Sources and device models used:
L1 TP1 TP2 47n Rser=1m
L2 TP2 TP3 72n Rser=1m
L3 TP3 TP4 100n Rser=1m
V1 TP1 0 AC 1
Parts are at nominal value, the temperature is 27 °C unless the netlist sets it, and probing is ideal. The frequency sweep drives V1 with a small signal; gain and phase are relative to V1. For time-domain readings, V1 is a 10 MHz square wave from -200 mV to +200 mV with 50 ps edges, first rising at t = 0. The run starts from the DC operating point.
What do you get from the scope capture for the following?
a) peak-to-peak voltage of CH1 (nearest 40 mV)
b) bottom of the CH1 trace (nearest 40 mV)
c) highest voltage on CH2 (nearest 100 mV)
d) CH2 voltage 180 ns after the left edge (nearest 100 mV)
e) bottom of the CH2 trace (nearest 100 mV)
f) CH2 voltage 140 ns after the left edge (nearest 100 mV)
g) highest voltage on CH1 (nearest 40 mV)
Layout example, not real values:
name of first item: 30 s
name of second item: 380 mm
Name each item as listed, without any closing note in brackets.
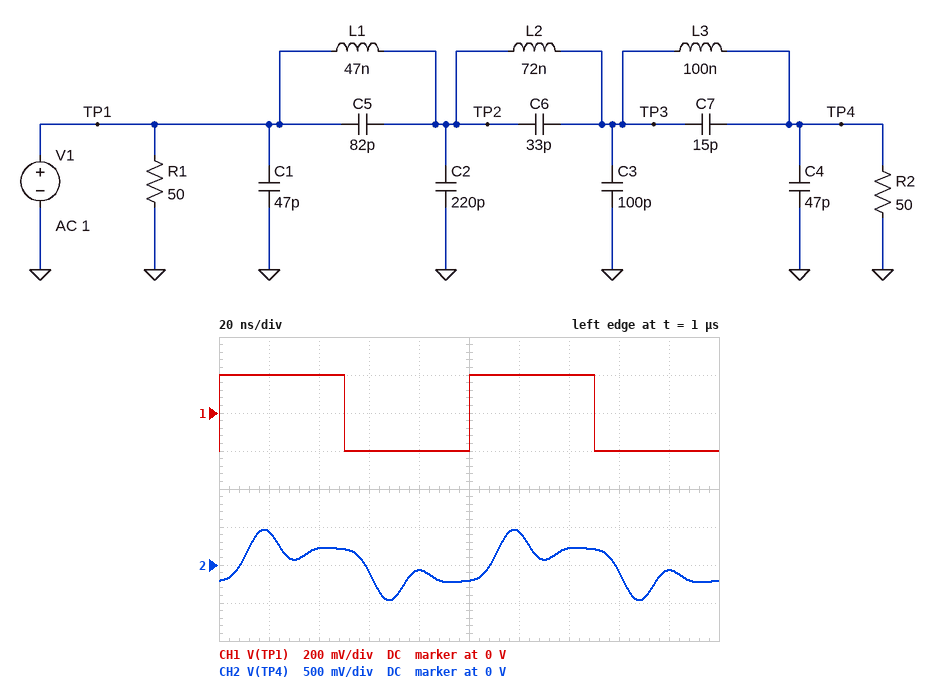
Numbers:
peak-to-peak voltage of CH1: 400 mV
bottom of the CH1 trace: -200 mV
highest voltage on CH2: 500 mV
CH2 voltage 180 ns after the left edge: -100 mV
bottom of the CH2 trace: -500 mV
CH2 voltage 140 ns after the left edge: 200 mV
highest voltage on CH1: 200 mV
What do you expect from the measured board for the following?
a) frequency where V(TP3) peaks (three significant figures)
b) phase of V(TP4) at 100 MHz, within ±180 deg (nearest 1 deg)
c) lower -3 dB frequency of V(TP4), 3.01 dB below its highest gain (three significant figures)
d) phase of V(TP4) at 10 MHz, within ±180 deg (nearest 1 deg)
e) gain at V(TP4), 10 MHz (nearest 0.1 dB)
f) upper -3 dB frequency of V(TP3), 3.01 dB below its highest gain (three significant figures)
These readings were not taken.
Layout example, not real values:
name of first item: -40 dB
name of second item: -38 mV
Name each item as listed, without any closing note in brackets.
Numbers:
frequency where V(TP3) peaks: 33.3 MHz
phase of V(TP4) at 100 MHz, within ±180 deg: 42 deg
lower -3 dB frequency of V(TP4), 3.01 dB below its highest gain: 22.5 MHz
phase of V(TP4) at 10 MHz, within ±180 deg: -17 deg
gain at V(TP4), 10 MHz: 0.8 dB
upper -3 dB frequency of V(TP3), 3.01 dB below its highest gain: 47.9 MHz
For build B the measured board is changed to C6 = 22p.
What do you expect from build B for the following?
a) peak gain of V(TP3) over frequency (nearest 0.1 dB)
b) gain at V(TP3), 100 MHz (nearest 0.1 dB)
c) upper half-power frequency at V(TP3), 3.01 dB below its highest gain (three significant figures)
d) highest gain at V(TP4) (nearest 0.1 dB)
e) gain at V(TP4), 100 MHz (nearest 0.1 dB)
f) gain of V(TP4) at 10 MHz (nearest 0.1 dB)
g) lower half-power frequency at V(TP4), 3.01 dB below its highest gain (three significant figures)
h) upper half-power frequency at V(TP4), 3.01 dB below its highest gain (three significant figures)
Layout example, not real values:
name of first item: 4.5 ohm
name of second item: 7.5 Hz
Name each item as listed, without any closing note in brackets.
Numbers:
peak gain of V(TP3) over frequency: 6.3 dB
gain at V(TP3), 100 MHz: -33.4 dB
upper half-power frequency at V(TP3), 3.01 dB below its highest gain: 46.6 MHz
highest gain at V(TP4): 7.3 dB
gain at V(TP4), 100 MHz: -46.9 dB
gain of V(TP4) at 10 MHz: 0.8 dB
lower half-power frequency at V(TP4), 3.01 dB below its highest gain: 22.8 MHz
upper half-power frequency at V(TP4), 3.01 dB below its highest gain: 47.5 MHz
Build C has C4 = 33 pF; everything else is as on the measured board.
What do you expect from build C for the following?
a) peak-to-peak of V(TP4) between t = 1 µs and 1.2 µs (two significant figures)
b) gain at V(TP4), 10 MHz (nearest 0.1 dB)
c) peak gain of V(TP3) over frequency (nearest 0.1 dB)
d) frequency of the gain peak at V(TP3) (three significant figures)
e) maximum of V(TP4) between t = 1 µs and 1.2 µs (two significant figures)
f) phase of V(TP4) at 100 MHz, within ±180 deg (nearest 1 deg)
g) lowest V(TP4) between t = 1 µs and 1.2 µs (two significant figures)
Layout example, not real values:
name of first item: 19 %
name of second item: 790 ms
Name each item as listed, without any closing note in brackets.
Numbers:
peak-to-peak of V(TP4) between t = 1 µs and 1.2 µs: 890 mV
gain at V(TP4), 10 MHz: 0.7 dB
peak gain of V(TP3) over frequency: 7.3 dB
frequency of the gain peak at V(TP3): 35.5 MHz
maximum of V(TP4) between t = 1 µs and 1.2 µs: 450 mV
phase of V(TP4) at 100 MHz, within ±180 deg: 56 deg
lowest V(TP4) between t = 1 µs and 1.2 µs: -450 mV
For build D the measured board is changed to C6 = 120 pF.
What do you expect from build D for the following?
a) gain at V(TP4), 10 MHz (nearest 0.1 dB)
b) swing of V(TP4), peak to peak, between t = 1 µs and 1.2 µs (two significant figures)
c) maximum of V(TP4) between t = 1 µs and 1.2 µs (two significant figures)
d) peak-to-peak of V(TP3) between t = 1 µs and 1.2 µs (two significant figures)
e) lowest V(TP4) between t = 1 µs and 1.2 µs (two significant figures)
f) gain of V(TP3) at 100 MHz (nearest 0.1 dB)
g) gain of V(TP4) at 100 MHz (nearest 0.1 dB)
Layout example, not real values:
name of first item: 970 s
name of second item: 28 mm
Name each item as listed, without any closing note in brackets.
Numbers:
gain at V(TP4), 10 MHz: 0.8 dB
swing of V(TP4), peak to peak, between t = 1 µs and 1.2 µs: 760 mV
maximum of V(TP4) between t = 1 µs and 1.2 µs: 380 mV
peak-to-peak of V(TP3) between t = 1 µs and 1.2 µs: 730 mV
lowest V(TP4) between t = 1 µs and 1.2 µs: -380 mV
gain of V(TP3) at 100 MHz: -26.5 dB
gain of V(TP4) at 100 MHz: -39.9 dB
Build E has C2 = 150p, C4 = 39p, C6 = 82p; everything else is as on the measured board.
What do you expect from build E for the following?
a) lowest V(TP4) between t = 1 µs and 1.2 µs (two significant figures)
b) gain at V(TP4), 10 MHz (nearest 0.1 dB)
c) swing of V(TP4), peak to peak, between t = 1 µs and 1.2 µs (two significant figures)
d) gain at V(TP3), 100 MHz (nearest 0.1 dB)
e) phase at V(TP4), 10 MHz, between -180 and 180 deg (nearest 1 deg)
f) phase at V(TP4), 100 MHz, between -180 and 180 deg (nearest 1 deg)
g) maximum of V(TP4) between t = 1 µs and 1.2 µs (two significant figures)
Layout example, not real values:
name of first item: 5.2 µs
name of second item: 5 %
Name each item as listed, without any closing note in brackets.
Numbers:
lowest V(TP4) between t = 1 µs and 1.2 µs: -420 mV
gain at V(TP4), 10 MHz: 0.6 dB
swing of V(TP4), peak to peak, between t = 1 µs and 1.2 µs: 840 mV
gain at V(TP3), 100 MHz: -26.6 dB
phase at V(TP4), 10 MHz, between -180 and 180 deg: -17 deg
phase at V(TP4), 100 MHz, between -180 and 180 deg: -131 deg
maximum of V(TP4) between t = 1 µs and 1.2 µs: 420 mV
